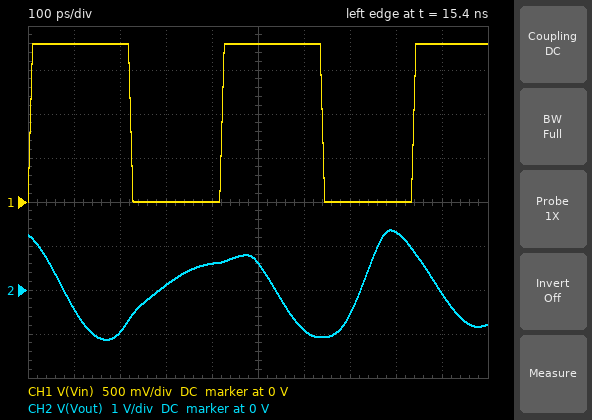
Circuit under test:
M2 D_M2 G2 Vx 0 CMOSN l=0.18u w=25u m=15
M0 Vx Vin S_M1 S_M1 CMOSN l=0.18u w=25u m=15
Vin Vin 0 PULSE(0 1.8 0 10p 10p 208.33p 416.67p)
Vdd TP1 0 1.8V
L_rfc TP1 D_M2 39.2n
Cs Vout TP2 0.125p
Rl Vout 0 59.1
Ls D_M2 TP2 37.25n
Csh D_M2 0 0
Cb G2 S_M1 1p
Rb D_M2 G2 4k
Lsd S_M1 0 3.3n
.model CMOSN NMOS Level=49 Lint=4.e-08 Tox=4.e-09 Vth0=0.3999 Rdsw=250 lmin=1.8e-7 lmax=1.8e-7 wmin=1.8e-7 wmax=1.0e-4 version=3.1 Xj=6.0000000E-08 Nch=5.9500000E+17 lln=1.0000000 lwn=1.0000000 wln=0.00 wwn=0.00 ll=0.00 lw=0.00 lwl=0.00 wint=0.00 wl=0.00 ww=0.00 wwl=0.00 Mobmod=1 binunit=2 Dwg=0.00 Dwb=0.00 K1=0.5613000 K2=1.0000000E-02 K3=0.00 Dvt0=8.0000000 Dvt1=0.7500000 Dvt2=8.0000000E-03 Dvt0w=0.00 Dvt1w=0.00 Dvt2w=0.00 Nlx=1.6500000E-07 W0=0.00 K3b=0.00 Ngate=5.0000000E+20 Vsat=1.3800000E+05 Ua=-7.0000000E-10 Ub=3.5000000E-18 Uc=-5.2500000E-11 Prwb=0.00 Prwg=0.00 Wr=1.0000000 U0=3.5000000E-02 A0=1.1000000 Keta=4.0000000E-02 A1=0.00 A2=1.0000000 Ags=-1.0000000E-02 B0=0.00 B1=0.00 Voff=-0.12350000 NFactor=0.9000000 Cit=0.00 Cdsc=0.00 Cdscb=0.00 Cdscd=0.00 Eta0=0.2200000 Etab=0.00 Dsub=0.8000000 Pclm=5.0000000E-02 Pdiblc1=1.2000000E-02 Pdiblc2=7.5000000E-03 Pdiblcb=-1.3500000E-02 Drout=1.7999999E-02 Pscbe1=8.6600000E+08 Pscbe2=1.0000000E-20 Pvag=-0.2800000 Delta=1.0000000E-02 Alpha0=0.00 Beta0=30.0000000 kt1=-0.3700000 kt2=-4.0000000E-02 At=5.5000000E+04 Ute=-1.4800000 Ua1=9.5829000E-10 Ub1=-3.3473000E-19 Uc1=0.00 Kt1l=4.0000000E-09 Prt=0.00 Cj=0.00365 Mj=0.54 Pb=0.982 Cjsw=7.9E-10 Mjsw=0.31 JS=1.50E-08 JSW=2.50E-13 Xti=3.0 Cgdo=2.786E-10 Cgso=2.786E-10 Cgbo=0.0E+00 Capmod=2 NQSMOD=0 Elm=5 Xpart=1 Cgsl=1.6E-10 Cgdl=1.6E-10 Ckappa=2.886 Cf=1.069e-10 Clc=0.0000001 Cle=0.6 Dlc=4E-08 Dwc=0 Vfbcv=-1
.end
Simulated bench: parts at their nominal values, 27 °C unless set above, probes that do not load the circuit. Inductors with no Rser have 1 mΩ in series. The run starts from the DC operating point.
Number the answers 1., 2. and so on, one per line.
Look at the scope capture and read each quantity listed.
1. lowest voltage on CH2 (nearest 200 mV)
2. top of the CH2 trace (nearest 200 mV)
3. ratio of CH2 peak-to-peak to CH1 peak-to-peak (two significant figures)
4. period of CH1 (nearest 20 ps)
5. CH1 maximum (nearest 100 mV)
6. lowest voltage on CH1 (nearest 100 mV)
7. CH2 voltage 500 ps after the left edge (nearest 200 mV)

1. -1.2 V
2. 1.4 V
3. 1.4
4. 420 ps
5. 1.8 V
6. 0 V
7. 600 mV
